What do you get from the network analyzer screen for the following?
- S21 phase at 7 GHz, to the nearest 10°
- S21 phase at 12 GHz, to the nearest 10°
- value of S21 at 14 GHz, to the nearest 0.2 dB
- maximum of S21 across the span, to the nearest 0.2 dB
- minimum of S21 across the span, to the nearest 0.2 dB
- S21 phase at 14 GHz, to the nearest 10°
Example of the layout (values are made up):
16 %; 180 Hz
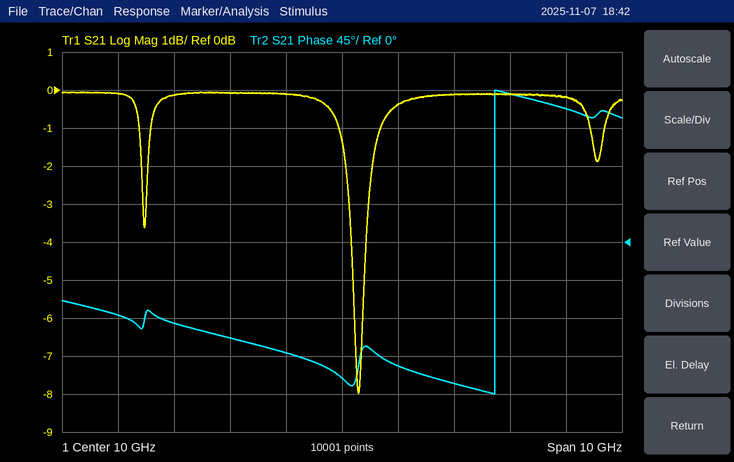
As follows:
-100°; -170°; -0.2 dB; 0.0 dB; -8.0 dB; 160°
